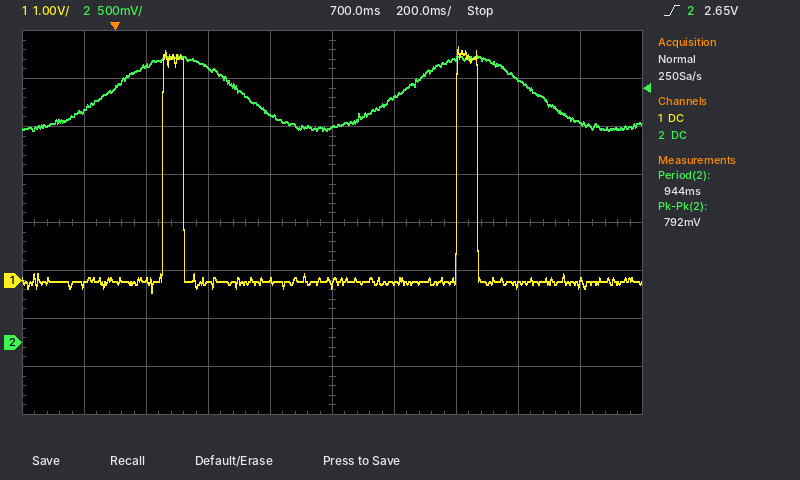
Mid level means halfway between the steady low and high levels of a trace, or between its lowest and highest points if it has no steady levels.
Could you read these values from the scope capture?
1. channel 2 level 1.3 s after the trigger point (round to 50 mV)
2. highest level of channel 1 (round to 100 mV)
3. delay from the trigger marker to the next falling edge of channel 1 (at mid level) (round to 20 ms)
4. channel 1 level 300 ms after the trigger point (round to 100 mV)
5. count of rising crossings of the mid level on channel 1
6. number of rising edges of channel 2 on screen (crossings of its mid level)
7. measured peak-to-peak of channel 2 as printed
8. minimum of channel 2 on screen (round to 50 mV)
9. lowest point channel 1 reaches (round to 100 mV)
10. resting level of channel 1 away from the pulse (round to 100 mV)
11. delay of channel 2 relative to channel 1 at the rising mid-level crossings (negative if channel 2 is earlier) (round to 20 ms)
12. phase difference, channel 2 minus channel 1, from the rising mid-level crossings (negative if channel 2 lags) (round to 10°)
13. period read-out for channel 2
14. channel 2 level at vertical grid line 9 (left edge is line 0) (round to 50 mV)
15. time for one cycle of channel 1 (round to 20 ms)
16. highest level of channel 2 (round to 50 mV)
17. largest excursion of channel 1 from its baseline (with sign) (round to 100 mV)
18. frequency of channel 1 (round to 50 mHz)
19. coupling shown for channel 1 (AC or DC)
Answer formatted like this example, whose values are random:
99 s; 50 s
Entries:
2.75 V; 4.9 V; 220 ms; -100 mV; 2; 2; 792 mV; 2.20 V; -300 mV; 0.0 V; -180 ms; +70°; 944 ms; 2.30 V; 940 ms; 3.00 V; +4.9 V; 1.05 Hz; DC
